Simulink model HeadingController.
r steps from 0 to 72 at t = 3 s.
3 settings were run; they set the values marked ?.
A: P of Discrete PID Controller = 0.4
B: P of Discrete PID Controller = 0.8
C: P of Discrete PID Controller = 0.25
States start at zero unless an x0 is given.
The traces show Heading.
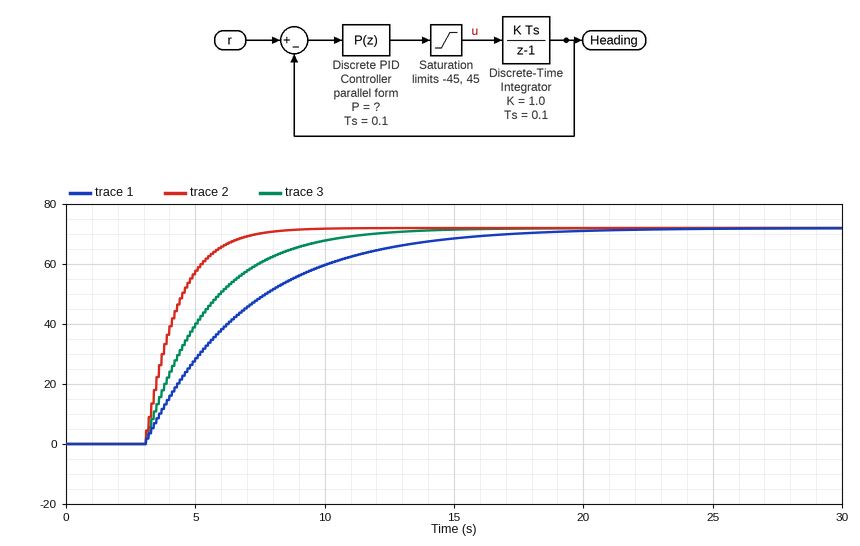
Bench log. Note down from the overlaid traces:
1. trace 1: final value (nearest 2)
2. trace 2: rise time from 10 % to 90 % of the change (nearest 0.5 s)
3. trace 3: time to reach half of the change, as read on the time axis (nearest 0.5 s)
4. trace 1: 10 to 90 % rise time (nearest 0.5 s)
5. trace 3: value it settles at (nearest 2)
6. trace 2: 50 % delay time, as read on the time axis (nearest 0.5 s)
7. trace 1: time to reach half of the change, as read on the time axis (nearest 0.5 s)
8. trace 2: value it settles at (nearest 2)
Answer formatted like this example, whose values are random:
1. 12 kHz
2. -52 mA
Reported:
1. 72
2. 2.5 s
3. 4.5 s
4. 8.5 s
5. 72
6. 4.0 s
7. 6.0 s
8. 72
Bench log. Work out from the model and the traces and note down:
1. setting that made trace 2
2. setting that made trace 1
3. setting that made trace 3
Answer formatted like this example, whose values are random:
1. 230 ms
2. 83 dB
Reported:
1. B
2. C
3. A
